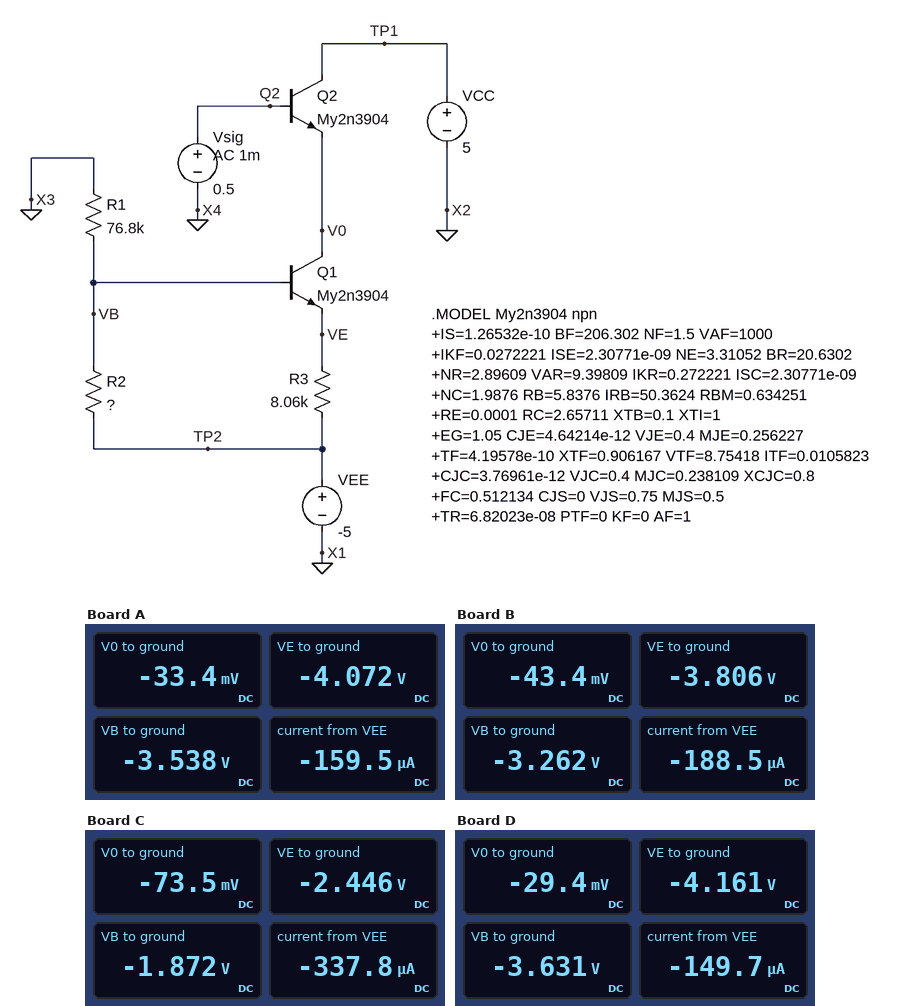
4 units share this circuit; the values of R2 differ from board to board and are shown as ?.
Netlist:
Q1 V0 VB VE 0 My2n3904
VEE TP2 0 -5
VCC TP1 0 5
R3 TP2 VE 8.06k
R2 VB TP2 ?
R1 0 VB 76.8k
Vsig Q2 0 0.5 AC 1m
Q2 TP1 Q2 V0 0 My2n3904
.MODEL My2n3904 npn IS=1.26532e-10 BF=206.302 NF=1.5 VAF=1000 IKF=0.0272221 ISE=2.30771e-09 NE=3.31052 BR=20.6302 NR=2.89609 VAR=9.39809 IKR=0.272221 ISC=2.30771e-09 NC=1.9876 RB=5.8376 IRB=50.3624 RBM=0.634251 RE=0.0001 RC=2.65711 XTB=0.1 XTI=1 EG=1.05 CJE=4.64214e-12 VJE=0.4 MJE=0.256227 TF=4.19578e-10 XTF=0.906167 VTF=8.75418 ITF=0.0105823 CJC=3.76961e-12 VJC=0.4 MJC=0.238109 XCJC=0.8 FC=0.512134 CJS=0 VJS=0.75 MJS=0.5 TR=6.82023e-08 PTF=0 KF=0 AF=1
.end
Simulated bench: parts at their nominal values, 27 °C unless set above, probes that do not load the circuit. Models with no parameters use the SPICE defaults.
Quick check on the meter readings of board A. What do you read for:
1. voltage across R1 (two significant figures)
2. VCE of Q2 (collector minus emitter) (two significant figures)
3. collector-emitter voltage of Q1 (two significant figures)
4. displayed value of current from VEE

3.5 V
5.0 V
4.0 V
-159.5 µA
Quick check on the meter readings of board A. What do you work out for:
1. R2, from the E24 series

33 kΩ
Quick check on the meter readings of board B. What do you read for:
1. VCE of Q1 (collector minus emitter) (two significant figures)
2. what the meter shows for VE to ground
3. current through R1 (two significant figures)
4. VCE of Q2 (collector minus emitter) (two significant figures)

3.8 V
-3.806 V
42 µA
5.0 V
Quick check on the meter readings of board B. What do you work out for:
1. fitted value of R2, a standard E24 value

43 kΩ
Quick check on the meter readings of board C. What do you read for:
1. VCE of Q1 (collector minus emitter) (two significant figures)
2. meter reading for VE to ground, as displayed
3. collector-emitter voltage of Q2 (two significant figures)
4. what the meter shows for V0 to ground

2.4 V
-2.446 V
5.1 V
-73.5 mV
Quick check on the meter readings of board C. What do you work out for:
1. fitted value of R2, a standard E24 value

150 kΩ
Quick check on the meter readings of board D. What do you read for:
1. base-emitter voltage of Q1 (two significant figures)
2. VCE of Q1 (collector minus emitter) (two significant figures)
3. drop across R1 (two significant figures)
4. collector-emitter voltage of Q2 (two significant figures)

530 mV
4.1 V
3.6 V
5.0 V
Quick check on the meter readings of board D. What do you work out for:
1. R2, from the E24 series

30 kΩ
